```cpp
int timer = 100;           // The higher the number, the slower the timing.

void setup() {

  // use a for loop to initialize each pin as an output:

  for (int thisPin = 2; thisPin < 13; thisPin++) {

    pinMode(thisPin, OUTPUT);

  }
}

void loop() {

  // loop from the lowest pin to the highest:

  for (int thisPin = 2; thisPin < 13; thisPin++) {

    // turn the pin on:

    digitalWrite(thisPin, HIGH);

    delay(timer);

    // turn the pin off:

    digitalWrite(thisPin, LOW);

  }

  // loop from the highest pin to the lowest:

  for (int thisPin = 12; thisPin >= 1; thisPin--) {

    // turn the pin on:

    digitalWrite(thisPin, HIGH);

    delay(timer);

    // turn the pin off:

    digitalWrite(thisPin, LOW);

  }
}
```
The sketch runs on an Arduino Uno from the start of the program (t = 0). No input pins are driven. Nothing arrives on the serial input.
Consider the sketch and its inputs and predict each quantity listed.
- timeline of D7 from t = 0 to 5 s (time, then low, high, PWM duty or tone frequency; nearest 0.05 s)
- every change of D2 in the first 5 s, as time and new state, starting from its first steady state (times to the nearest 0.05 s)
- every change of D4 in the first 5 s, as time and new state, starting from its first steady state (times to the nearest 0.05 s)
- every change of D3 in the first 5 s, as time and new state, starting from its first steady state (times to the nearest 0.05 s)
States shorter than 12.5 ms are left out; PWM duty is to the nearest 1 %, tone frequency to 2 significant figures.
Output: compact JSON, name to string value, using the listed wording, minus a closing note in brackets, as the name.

{"timeline of D7 from t = 0 to 5 s": "0 s low; 0.5 s high; 0.6 s low; 1.6 s high; 1.7 s low; 2.8 s high; 2.9 s low; 3.9 s high; 4 s low", "every change of D2 in the first 5 s, as time and new state, starting from its first steady state": "0 s high; 0.1 s low; 2.1 s high; 2.2 s low; 2.3 s high; 2.4 s low; 4.4 s high; 4.5 s low; 4.6 s high; 4.7 s low", "every change of D4 in the first 5 s, as time and new state, starting from its first steady state": "0 s low; 0.2 s high; 0.3 s low; 1.9 s high; 2 s low; 2.5 s high; 2.6 s low; 4.2 s high; 4.3 s low; 4.8 s high; 4.9 s low", "every change of D3 in the first 5 s, as time and new state, starting from its first steady state": "0 s low; 0.1 s high; 0.2 s low; 2 s high; 2.1 s low; 2.4 s high; 2.5 s low; 4.3 s high; 4.4 s low; 4.7 s high; 4.8 s low"}
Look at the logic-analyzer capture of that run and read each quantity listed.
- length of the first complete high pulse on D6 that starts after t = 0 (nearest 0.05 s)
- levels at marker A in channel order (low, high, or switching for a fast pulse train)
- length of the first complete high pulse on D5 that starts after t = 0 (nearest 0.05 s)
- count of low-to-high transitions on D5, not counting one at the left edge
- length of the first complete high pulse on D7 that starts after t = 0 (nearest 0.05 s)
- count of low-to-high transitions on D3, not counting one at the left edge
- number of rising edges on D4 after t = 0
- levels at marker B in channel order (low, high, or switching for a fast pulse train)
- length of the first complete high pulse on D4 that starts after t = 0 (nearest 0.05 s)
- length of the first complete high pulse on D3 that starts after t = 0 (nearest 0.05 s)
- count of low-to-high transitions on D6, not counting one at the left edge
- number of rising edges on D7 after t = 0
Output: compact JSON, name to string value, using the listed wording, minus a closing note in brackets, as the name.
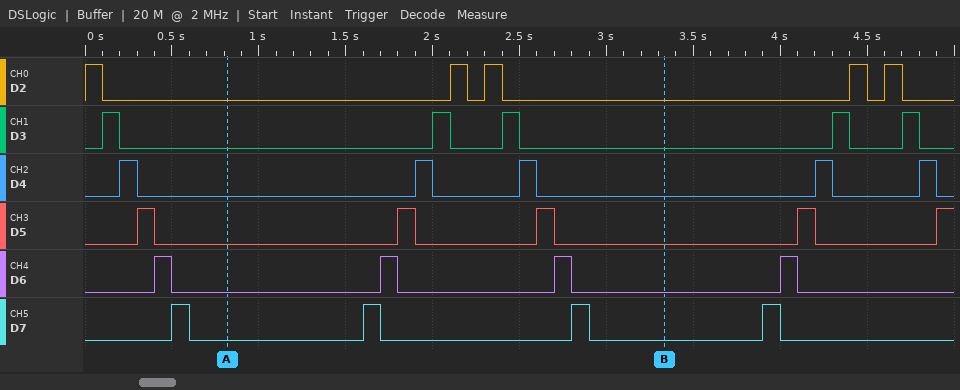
{"length of the first complete high pulse on D6 that starts after t = 0": "0.10 s", "levels at marker A in channel order": "D2 low, D3 low, D4 low, D5 low, D6 low, D7 low", "length of the first complete high pulse on D5 that starts after t = 0": "0.10 s", "count of low-to-high transitions on D5, not counting one at the left edge": "5", "length of the first complete high pulse on D7 that starts after t = 0": "0.10 s", "count of low-to-high transitions on D3, not counting one at the left edge": "5", "number of rising edges on D4 after t = 0": "5", "levels at marker B in channel order": "D2 low, D3 low, D4 low, D5 low, D6 low, D7 low", "length of the first complete high pulse on D4 that starts after t = 0": "0.10 s", "length of the first complete high pulse on D3 that starts after t = 0": "0.10 s", "count of low-to-high transitions on D6, not counting one at the left edge": "4", "number of rising edges on D7 after t = 0": "4"}
